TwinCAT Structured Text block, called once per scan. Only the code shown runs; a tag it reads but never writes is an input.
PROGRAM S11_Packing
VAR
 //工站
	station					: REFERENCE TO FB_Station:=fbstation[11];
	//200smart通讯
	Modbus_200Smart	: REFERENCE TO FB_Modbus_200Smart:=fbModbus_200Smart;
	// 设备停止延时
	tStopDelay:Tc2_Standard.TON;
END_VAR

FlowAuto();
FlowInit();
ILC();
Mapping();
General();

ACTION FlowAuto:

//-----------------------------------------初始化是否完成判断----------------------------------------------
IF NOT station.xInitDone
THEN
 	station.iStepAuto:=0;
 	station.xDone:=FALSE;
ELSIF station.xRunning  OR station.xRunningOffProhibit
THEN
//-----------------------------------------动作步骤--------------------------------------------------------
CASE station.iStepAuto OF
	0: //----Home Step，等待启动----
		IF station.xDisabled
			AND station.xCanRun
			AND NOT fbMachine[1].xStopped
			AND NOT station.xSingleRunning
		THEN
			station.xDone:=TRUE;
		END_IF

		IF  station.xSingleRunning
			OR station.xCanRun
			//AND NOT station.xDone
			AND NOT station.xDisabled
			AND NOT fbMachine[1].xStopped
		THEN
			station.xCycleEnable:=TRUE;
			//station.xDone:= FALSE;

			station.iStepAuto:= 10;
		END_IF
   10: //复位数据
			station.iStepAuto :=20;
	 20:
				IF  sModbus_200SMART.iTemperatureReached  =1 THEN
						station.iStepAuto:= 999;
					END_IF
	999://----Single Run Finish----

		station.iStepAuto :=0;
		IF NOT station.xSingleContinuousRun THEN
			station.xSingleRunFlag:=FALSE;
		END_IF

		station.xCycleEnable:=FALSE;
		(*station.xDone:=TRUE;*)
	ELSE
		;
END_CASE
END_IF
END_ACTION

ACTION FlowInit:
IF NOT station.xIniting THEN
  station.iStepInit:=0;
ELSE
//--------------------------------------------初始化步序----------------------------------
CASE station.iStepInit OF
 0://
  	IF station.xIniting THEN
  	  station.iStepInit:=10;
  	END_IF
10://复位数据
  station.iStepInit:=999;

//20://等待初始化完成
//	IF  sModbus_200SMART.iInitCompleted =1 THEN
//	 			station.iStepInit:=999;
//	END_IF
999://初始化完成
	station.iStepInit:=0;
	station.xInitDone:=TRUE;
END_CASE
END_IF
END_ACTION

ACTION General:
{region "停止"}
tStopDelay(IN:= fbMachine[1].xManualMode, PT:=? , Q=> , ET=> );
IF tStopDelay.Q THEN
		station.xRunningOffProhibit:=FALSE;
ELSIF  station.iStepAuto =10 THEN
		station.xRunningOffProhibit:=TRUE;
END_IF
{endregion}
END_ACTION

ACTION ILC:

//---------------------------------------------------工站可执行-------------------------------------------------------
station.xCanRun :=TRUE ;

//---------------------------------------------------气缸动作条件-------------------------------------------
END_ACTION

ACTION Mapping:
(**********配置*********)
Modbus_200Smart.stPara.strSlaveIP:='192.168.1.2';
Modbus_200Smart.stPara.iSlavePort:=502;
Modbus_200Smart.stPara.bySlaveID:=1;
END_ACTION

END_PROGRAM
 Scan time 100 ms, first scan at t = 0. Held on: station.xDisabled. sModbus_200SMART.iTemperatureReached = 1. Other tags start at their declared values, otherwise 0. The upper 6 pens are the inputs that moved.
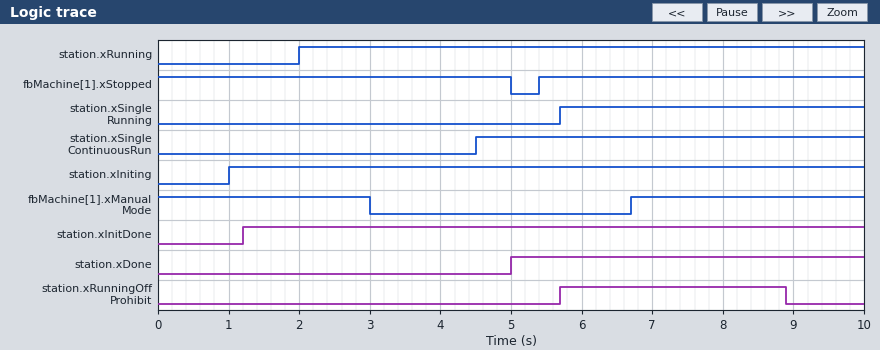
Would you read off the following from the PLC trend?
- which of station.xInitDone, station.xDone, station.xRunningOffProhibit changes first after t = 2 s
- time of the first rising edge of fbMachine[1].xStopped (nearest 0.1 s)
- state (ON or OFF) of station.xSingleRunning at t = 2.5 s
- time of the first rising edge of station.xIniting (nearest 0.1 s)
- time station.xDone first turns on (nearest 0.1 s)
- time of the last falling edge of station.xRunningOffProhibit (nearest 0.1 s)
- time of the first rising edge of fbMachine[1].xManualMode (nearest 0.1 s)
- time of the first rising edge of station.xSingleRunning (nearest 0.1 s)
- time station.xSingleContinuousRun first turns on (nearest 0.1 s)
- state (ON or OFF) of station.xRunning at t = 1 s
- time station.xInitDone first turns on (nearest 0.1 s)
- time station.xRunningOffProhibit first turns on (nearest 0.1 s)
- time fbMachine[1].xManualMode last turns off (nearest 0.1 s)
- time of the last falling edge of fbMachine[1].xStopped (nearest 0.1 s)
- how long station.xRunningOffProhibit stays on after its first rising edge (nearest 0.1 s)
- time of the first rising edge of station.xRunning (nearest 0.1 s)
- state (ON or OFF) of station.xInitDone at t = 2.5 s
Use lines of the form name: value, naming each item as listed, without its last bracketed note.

which of station.xInitDone, station.xDone, station.xRunningOffProhibit changes first after t = 2 s: station.xDone
time of the first rising edge of fbMachine[1].xStopped: 5.4 s
state (ON or OFF) of station.xSingleRunning at t = 2.5 s: OFF
time of the first rising edge of station.xIniting: 1.0 s
time station.xDone first turns on: 5.0 s
time of the last falling edge of station.xRunningOffProhibit: 8.9 s
time of the first rising edge of fbMachine[1].xManualMode: 6.7 s
time of the first rising edge of station.xSingleRunning: 5.7 s
time station.xSingleContinuousRun first turns on: 4.5 s
state (ON or OFF) of station.xRunning at t = 1 s: OFF
time station.xInitDone first turns on: 1.2 s
time station.xRunningOffProhibit first turns on: 5.7 s
time fbMachine[1].xManualMode last turns off: 3.0 s
time of the last falling edge of fbMachine[1].xStopped: 5.0 s
how long station.xRunningOffProhibit stays on after its first rising edge: 3.2 s
time of the first rising edge of station.xRunning: 2.0 s
state (ON or OFF) of station.xInitDone at t = 2.5 s: ON
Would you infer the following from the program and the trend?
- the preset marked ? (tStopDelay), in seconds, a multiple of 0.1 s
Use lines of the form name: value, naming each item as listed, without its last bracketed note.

the preset marked ? (tStopDelay), in seconds, a multiple of 0.1 s: 2.2 s
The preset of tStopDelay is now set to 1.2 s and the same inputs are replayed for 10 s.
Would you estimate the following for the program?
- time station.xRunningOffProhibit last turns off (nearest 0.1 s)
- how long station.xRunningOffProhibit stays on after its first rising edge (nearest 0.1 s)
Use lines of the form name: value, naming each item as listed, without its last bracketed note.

time station.xRunningOffProhibit last turns off: 7.9 s
how long station.xRunningOffProhibit stays on after its first rising edge: 2.2 s
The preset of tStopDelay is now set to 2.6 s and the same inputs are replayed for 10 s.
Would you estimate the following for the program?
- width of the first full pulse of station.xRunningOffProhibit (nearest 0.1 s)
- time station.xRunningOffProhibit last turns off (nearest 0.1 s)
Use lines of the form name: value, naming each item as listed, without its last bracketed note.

width of the first full pulse of station.xRunningOffProhibit: 3.6 s
time station.xRunningOffProhibit last turns off: 9.3 s
